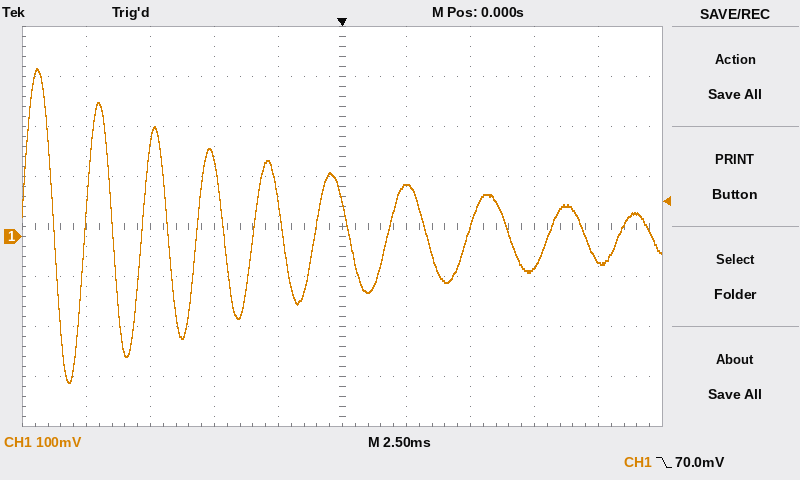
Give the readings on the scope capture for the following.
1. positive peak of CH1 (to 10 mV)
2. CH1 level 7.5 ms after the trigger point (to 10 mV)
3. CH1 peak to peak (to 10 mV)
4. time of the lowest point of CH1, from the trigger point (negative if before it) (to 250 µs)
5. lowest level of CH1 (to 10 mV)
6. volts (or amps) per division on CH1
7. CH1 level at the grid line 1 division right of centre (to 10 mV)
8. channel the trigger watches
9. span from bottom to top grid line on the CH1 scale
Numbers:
340 mV
-60 mV
630 mV
-10.75 ms
-290 mV
100 mV
100 mV
CH1
800 mV
